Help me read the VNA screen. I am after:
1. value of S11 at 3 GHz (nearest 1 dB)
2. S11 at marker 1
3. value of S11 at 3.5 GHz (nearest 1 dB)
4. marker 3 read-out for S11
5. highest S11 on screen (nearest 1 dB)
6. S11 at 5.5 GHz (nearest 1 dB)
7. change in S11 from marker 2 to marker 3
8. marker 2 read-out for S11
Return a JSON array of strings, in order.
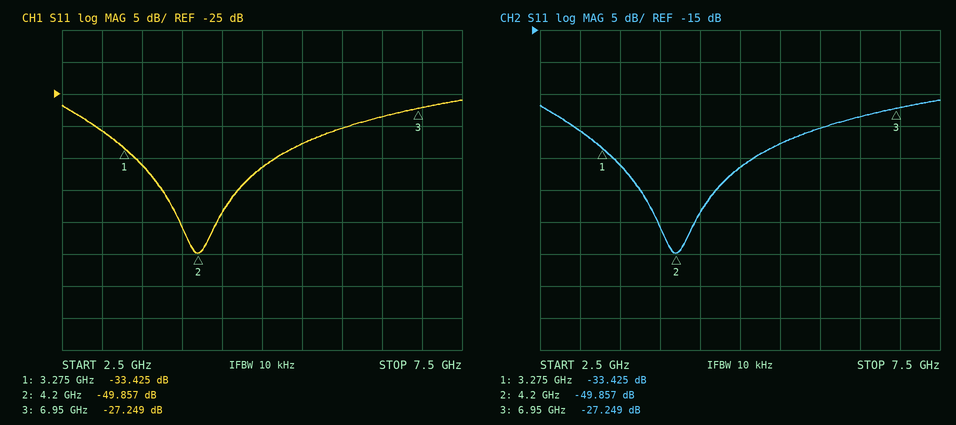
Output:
["-31 dB", "-33.425 dB", "-36 dB", "-27.249 dB", "-26 dB", "-33 dB", "22.608 dB", "-49.857 dB"]
